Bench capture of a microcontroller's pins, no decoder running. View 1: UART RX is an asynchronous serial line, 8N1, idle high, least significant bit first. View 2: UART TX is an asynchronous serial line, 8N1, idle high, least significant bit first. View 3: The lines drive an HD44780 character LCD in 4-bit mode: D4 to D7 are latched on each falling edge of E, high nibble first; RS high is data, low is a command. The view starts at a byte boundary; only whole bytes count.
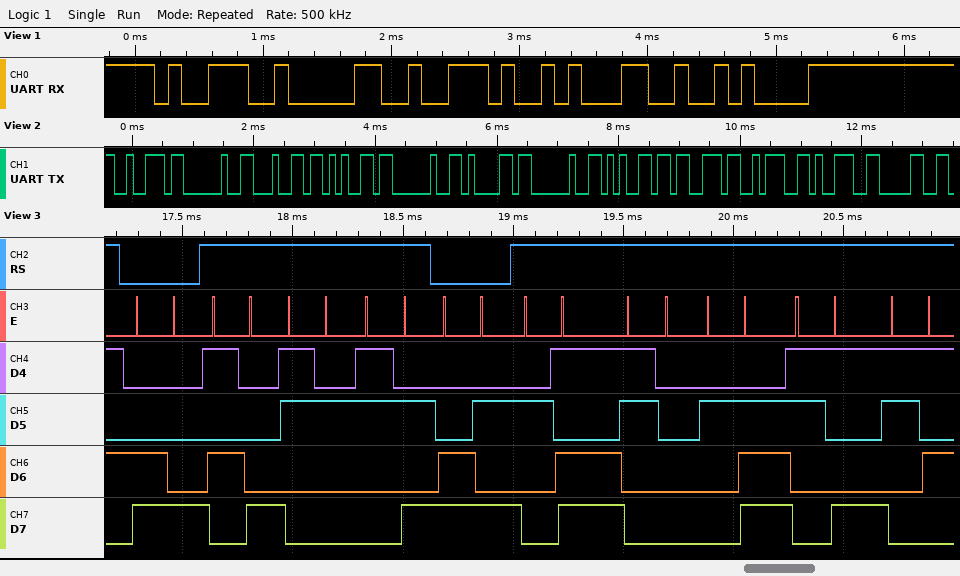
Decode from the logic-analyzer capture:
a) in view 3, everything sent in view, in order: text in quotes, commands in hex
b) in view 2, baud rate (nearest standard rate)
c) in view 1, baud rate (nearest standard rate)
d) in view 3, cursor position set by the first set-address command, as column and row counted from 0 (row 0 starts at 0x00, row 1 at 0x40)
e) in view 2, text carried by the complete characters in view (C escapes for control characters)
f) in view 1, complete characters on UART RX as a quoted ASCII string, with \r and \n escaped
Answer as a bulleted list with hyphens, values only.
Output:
- 0xC8 "X2:" 0xCA "-0.95"
- 9600 baud
- 9600 baud
- column 8, row 1
- "r de a es:90"
- "90.1\n"
